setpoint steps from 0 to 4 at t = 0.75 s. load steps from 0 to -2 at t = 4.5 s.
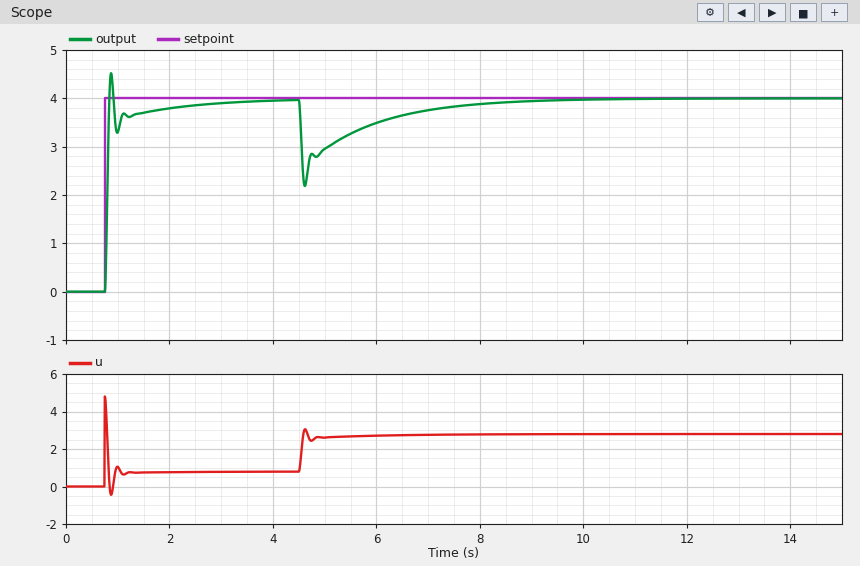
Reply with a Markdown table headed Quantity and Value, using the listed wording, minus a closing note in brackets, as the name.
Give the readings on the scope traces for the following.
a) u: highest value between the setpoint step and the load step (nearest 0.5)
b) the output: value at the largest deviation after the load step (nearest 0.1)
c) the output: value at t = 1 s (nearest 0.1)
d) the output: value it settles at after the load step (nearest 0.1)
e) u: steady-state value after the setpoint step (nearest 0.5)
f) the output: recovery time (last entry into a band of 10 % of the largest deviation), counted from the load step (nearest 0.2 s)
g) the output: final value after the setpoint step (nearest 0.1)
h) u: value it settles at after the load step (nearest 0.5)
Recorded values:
| Quantity | Value |
|---|---|
| u: highest value between the setpoint step and the load step | 5.0 |
| the output: value at the largest deviation after the load step | 2.2 |
| the output: value at t = 1 s | 3.3 |
| the output: value it settles at after the load step | 4.0 |
| u: steady-state value after the setpoint step | 1.0 |
| the output: recovery time (last entry into a band of 10 % of the largest deviation), counted from the load step | 3.0 s |
| the output: final value after the setpoint step | 4.0 |
| u: value it settles at after the load step | 3.0 |
